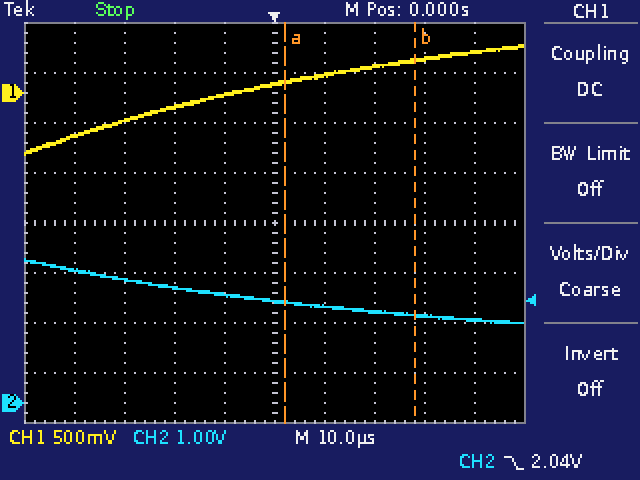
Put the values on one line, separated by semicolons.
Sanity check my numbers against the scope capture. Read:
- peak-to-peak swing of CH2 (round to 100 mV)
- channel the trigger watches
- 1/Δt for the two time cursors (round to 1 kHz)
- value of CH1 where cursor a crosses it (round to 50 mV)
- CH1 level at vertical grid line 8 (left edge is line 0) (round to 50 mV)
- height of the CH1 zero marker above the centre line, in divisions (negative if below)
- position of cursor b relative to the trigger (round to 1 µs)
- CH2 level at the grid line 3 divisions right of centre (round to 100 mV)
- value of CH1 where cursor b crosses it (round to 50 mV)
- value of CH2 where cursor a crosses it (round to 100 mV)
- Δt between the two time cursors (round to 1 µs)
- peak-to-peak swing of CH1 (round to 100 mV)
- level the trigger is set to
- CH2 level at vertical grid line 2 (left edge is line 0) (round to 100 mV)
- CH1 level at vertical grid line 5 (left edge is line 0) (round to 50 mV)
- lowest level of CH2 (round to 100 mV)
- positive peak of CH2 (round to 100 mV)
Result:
1.3 V; CH2; 38 kHz; 100 mV; 350 mV; +2.6 div; +28 µs; 1.7 V; 300 mV; 2.0 V; 26 µs; 1.10 V; 2.04 V; 2.5 V; 100 mV; 1.6 V; 2.9 V
